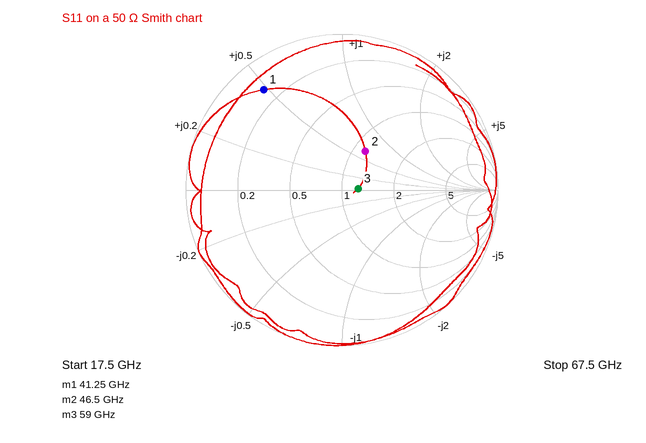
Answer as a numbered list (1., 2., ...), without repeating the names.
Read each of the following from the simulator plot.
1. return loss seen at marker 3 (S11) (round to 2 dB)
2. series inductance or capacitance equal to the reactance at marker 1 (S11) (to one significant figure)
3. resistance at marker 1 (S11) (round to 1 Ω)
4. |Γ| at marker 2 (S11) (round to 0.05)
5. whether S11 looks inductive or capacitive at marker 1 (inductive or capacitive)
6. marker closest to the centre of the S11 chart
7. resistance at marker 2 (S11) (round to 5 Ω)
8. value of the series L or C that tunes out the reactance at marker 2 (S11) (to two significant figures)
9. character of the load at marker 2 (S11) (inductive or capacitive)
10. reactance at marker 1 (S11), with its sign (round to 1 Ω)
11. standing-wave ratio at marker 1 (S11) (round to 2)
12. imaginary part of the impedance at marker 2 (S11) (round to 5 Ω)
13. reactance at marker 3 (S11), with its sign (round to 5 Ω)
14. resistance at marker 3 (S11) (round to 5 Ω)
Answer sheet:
1. 20 dB
2. 90 pH
3. 6 Ω
4. 0.30
5. inductive
6. marker 3
7. 60 Ω
8. 110 fF
9. inductive
10. +24 Ω
11. 10
12. +30 Ω
13. 0 Ω
14. 60 Ω
